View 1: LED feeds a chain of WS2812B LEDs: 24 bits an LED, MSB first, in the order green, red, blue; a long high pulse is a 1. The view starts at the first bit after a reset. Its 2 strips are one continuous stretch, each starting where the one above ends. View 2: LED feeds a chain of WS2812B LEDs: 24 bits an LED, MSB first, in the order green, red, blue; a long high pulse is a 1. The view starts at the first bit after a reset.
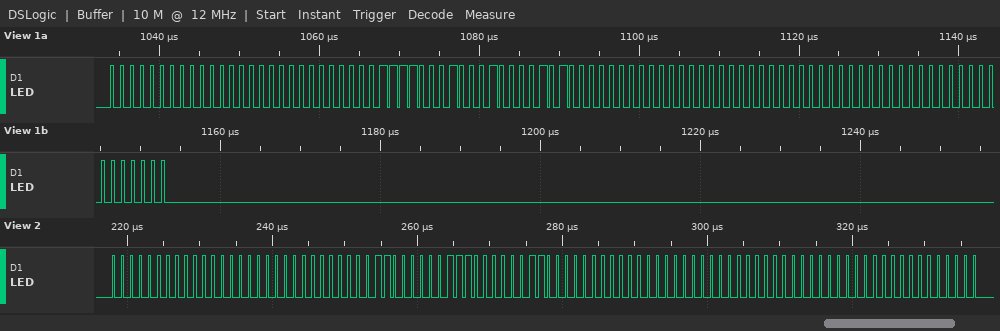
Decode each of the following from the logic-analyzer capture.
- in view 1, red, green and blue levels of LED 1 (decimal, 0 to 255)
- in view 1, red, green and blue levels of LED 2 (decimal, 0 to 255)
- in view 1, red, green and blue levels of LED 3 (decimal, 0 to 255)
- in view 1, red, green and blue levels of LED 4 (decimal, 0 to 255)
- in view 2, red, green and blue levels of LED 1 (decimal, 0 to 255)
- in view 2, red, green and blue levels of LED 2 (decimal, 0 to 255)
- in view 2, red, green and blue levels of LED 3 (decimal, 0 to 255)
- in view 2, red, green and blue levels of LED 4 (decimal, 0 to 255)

0, 0, 0
34, 30, 20
0, 0, 0
0, 0, 0
0, 0, 0
7, 6, 3
0, 0, 0
0, 0, 0
